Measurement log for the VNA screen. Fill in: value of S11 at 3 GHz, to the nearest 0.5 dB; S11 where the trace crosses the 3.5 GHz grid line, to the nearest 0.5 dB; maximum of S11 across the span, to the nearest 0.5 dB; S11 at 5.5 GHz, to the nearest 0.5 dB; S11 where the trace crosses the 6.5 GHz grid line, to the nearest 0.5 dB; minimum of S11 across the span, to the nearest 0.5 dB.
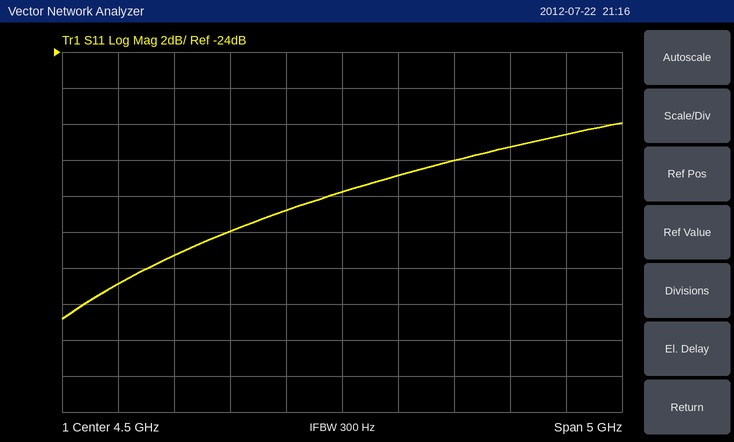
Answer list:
-35.5 dB
-34.0 dB
-28.0 dB
-30.0 dB
-28.5 dB
-39.0 dB
